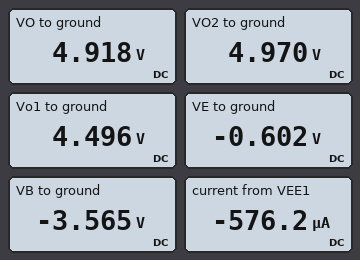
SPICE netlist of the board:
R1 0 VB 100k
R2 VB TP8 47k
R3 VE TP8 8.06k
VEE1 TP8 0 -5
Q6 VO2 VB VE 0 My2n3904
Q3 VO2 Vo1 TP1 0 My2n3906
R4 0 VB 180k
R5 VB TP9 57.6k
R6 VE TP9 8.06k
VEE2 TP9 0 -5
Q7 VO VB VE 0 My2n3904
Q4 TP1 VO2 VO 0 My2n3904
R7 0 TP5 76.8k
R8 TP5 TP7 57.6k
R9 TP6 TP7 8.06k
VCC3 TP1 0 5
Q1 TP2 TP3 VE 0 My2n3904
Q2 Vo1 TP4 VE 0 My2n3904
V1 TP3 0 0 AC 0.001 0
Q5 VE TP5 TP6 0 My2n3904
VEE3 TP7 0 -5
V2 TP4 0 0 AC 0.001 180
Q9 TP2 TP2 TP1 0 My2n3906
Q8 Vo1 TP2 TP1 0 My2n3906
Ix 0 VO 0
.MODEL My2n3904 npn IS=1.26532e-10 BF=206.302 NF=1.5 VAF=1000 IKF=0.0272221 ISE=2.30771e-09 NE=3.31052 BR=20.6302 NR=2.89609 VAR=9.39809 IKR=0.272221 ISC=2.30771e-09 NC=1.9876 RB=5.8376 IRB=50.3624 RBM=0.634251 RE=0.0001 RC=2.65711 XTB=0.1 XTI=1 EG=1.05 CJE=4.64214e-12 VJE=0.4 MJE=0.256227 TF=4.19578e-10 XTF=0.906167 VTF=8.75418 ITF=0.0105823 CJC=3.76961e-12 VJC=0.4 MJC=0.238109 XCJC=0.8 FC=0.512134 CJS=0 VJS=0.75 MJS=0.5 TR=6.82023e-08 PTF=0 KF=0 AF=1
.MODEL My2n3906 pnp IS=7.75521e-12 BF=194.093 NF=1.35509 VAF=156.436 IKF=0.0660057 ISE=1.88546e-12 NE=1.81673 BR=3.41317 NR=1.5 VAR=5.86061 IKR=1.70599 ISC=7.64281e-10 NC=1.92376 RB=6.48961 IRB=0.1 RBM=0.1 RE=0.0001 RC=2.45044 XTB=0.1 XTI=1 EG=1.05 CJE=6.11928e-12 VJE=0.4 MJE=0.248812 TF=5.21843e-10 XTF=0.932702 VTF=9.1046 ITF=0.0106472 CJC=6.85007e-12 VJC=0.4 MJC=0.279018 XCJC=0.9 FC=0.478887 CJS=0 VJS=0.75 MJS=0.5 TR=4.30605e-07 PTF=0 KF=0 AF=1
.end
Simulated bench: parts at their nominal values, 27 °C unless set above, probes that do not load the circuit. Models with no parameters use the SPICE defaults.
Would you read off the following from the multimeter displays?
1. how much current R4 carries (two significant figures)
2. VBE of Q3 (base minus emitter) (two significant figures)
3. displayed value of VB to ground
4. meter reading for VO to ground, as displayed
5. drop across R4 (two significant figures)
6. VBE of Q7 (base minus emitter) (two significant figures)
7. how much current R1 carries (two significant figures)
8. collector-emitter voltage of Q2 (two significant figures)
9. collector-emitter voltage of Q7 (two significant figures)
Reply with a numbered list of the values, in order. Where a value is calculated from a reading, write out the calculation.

1. (0 V - (-3.565 V)) / 180 kΩ = 20 µA
2. 4.496 V - 5 V = -500 mV
3. -3.565 V
4. 4.918 V
5. 0 V - (-3.565 V) = 3.6 V
6. -3.565 V - (-602 mV) = -3.0 V
7. (0 V - (-3.565 V)) / 100 kΩ = 36 µA
8. 4.496 V - (-602 mV) = 5.1 V
9. 4.918 V - (-602 mV) = 5.5 V
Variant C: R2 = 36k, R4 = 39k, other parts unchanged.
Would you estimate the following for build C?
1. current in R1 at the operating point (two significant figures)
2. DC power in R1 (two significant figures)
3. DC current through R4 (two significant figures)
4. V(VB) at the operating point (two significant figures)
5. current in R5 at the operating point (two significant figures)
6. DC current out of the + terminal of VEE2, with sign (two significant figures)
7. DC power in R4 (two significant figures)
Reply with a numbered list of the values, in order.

1. 28 µA
2. 78 µW
3. 72 µA
4. -2.8 V
5. 38 µA
6. -580 µA
7. 200 µW
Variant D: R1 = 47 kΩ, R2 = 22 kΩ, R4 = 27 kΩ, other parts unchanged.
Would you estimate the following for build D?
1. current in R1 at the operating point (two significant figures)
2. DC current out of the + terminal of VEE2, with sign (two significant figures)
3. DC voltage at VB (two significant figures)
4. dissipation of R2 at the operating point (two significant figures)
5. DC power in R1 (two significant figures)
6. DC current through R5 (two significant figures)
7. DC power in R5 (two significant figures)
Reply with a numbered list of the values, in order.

1. 55 µA
2. -590 µA
3. -2.6 V
4. 260 µW
5. 140 µW
6. 42 µA
7. 100 µW
